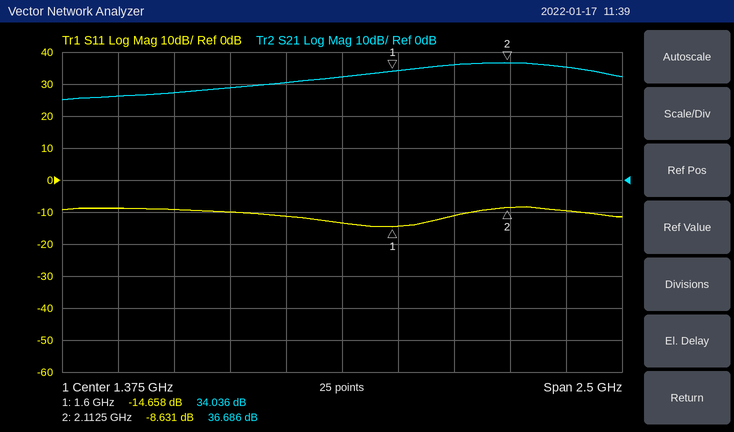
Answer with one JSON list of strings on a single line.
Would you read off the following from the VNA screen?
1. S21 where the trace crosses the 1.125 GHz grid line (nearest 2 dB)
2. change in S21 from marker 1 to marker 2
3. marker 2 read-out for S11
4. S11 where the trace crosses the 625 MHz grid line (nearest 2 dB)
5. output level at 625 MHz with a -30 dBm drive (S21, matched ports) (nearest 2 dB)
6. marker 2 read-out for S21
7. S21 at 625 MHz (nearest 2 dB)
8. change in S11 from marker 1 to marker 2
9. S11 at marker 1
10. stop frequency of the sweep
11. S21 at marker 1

["30 dB", "2.650 dB", "-8.631 dB", "-10 dB", "-2 dBm", "36.686 dB", "28 dB", "6.027 dB", "-14.658 dB", "2.625 GHz", "34.036 dB"]
